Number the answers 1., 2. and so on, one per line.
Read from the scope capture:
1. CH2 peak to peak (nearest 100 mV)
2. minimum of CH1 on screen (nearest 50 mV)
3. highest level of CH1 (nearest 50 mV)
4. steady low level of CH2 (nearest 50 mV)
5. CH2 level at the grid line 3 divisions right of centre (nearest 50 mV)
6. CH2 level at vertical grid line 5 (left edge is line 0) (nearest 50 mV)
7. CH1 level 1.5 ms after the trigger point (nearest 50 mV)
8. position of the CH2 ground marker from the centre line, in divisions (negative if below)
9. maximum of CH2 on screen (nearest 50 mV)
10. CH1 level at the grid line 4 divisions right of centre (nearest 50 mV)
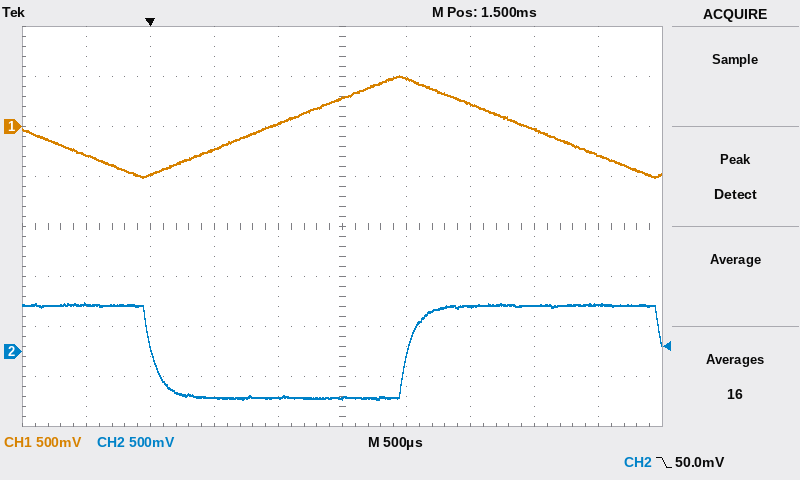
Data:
1. 1.00 V
2. -500 mV
3. 500 mV
4. -450 mV
5. 450 mV
6. -450 mV
7. 300 mV
8. -2.5 div
9. 500 mV
10. -300 mV
